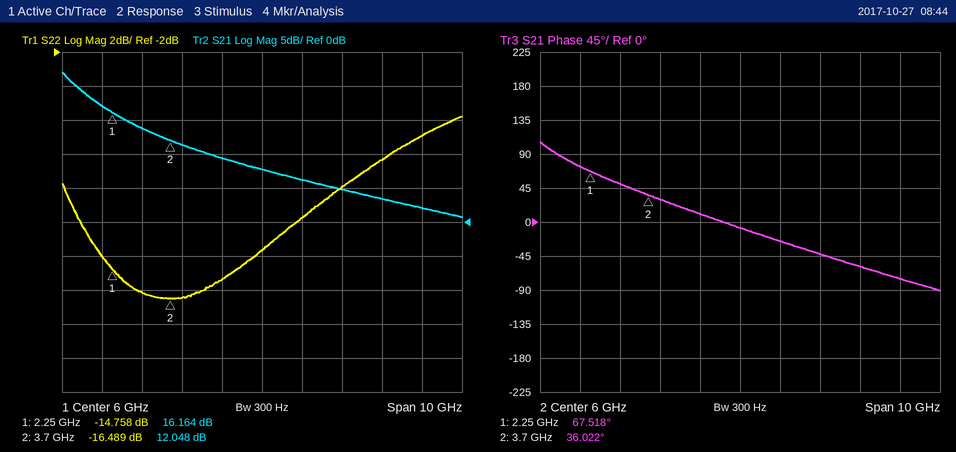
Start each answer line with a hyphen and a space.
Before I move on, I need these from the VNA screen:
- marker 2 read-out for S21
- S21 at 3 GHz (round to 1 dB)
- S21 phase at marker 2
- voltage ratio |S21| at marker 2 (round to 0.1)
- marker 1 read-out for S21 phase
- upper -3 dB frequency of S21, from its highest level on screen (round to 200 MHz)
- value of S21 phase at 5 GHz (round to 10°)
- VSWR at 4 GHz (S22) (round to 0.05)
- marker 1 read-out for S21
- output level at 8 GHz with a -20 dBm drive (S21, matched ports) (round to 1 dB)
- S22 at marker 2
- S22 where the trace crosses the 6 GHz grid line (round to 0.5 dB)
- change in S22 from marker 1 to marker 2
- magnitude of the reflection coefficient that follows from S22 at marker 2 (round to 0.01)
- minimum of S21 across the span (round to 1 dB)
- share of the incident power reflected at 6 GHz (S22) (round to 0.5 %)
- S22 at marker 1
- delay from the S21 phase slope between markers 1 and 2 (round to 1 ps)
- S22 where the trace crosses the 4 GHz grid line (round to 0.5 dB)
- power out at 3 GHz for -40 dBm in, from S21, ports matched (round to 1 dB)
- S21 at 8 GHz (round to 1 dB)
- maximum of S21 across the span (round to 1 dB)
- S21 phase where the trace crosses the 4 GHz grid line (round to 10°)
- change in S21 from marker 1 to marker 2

- 12.048 dB
- 14 dB
- 36.022°
- 4.0
- 67.518°
- 1.6 GHz
- 10°
- 1.35
- 16.164 dB
- -15 dBm
- -16.489 dB
- -13.5 dB
- -1.731 dB
- 0.15
- 1 dB
- 4.5 %
- -14.758 dB
- 60 ps
- -16.5 dB
- -26 dBm
- 5 dB
- 22 dB
- 30°
- -4.116 dB
